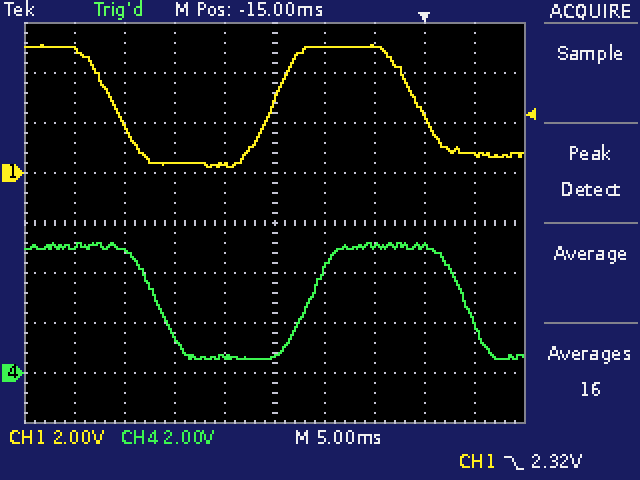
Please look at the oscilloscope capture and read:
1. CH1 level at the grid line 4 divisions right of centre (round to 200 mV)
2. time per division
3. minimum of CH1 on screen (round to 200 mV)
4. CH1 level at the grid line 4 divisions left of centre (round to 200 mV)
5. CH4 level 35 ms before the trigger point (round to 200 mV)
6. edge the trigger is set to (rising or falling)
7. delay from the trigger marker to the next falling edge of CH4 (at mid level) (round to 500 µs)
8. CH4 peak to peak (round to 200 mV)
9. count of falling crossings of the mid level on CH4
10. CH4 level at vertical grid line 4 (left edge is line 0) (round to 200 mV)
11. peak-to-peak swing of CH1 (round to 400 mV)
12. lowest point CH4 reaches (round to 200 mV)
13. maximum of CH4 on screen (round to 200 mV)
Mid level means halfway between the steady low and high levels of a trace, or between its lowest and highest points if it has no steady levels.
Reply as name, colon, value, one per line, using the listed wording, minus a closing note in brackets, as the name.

CH1 level at the grid line 4 divisions right of centre: 800 mV
time per division: 5 ms
minimum of CH1 on screen: 200 mV
CH1 level at the grid line 4 divisions left of centre: 5.0 V
CH4 level 35 ms before the trigger point: 5.0 V
edge the trigger is set to: falling
delay from the trigger marker to the next falling edge of CH4 (at mid level): 4.0 ms
CH4 peak to peak: 4.6 V
count of falling crossings of the mid level on CH4: 2
CH4 level at vertical grid line 4 (left edge is line 0): 600 mV
peak-to-peak swing of CH1: 4.8 V
lowest point CH4 reaches: 600 mV
maximum of CH4 on screen: 5.2 V
